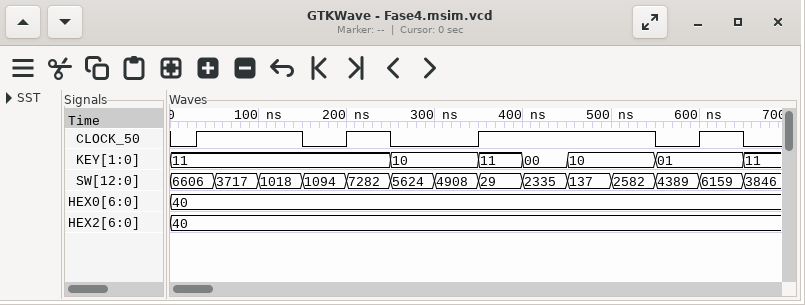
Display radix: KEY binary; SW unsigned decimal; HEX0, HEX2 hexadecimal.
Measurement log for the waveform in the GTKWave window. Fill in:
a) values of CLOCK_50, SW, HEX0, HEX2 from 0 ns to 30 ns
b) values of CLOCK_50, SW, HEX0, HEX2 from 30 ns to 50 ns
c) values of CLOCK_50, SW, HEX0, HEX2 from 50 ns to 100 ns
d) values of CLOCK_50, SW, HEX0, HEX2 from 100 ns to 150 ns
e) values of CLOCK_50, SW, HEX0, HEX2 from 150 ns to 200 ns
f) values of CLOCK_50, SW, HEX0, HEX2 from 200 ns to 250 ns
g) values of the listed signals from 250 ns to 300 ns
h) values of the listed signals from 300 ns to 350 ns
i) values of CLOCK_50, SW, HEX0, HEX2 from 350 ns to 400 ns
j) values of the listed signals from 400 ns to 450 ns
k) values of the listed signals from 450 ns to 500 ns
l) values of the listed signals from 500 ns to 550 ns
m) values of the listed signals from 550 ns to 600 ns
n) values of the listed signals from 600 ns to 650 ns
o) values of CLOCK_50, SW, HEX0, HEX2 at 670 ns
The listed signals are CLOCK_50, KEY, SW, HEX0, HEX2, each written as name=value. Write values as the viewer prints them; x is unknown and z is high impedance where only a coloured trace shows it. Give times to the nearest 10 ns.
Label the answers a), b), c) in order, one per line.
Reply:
a) CLOCK_50=0, SW=6606, HEX0=40, HEX2=40
b) CLOCK_50=1, SW=6606, HEX0=40, HEX2=40
c) CLOCK_50=1, SW=3717, HEX0=40, HEX2=40
d) CLOCK_50=1, SW=1018, HEX0=40, HEX2=40
e) CLOCK_50=0, SW=1094, HEX0=40, HEX2=40
f) CLOCK_50=1, SW=7282, HEX0=40, HEX2=40
g) CLOCK_50=0, KEY=10, SW=5624, HEX0=40, HEX2=40
h) CLOCK_50=0, KEY=10, SW=4908, HEX0=40, HEX2=40
i) CLOCK_50=1, SW=29, HEX0=40, HEX2=40
j) CLOCK_50=1, KEY=00, SW=2335, HEX0=40, HEX2=40
k) CLOCK_50=1, KEY=10, SW=137, HEX0=40, HEX2=40
l) CLOCK_50=1, KEY=10, SW=2582, HEX0=40, HEX2=40
m) CLOCK_50=0, KEY=01, SW=4389, HEX0=40, HEX2=40
n) CLOCK_50=1, KEY=01, SW=6159, HEX0=40, HEX2=40
o) CLOCK_50=0, SW=3846, HEX0=40, HEX2=40
